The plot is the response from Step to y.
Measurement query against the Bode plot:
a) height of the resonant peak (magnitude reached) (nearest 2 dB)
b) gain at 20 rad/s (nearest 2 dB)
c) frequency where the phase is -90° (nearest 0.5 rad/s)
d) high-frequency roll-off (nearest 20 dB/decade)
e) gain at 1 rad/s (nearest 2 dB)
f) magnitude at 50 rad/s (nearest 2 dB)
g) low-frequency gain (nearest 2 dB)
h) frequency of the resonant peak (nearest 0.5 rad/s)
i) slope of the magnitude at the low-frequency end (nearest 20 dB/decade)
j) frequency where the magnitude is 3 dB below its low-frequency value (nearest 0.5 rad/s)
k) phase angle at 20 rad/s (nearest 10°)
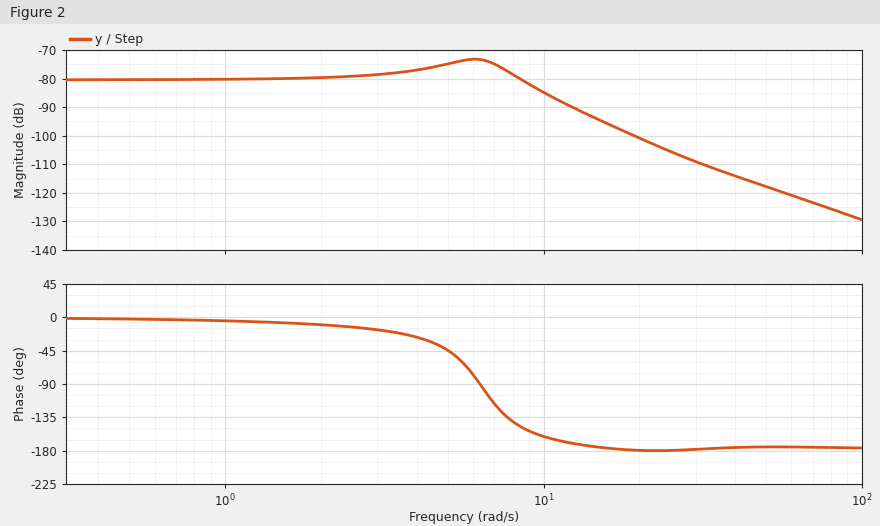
-74 dB
-100 dB
6.5 rad/s
-40 dB/decade
-80 dB
-118 dB
-80 dB
6.0 rad/s
0 dB/decade
9.5 rad/s
-180°
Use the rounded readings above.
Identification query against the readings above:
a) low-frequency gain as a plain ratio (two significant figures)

0.00010
